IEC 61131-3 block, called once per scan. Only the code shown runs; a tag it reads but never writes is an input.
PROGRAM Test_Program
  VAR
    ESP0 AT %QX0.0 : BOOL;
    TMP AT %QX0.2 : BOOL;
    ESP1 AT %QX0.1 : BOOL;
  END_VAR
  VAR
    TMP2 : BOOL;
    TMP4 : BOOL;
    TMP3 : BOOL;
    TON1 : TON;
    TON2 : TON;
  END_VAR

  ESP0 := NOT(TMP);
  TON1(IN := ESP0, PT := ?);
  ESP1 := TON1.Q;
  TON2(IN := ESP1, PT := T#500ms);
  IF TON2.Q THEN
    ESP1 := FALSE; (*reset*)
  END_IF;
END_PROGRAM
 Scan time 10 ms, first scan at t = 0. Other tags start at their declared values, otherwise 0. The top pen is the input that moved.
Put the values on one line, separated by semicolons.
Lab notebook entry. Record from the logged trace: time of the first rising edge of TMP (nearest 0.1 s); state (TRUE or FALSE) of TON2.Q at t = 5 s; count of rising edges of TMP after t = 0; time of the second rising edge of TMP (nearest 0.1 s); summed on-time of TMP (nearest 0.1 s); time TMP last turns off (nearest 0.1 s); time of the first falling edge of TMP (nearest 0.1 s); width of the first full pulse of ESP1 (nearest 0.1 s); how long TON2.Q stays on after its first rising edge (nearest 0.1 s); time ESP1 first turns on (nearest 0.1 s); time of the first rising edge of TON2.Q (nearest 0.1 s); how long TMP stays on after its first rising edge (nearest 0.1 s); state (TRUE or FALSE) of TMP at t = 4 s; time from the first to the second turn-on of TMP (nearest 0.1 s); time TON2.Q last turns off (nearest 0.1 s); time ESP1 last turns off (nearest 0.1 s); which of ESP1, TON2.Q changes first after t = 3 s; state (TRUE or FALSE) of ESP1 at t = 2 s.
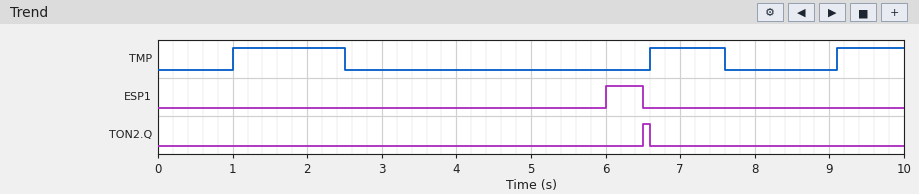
1.0 s; FALSE; 3; 6.6 s; 3.4 s; 7.6 s; 2.5 s; 0.5 s; 0.1 s; 6.0 s; 6.5 s; 1.5 s; FALSE; 5.6 s; 6.6 s; 6.5 s; ESP1; FALSE
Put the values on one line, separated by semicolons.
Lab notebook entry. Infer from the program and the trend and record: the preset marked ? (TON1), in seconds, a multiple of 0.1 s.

3.5 s
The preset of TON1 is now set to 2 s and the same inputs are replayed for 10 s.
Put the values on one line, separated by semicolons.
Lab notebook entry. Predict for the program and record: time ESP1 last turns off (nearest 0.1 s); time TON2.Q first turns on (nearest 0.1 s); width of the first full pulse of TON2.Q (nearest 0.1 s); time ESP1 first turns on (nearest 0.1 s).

5.0 s; 5.0 s; 1.6 s; 4.5 s
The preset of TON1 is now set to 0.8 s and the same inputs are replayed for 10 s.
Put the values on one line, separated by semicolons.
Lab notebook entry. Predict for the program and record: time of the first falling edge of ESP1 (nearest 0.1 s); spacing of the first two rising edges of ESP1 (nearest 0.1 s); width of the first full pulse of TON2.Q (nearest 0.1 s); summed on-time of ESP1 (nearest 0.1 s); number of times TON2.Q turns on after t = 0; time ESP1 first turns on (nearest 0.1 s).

1.0 s; 2.5 s; 2.8 s; 1.2 s; 2; 0.8 s
